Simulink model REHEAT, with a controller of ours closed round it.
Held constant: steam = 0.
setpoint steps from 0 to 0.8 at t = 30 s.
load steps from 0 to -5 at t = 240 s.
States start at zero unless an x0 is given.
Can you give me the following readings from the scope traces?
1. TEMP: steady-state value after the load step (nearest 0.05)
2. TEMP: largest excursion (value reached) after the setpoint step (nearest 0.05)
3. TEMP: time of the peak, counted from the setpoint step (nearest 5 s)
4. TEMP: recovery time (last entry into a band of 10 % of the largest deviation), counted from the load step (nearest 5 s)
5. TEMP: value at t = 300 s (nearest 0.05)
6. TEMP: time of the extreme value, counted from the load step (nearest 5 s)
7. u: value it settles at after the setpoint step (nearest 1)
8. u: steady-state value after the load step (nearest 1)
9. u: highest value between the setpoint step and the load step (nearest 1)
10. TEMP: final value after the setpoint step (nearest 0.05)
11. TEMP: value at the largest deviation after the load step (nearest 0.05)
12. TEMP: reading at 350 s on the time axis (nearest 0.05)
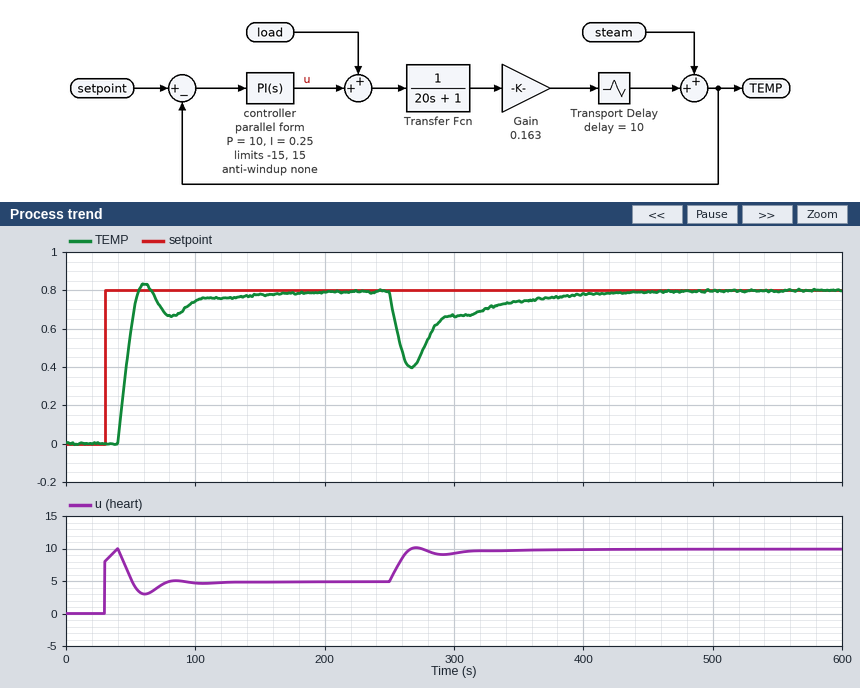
0.80
0.85
30 s
130 s
0.65
25 s
5
10
10
0.80
0.40
0.75
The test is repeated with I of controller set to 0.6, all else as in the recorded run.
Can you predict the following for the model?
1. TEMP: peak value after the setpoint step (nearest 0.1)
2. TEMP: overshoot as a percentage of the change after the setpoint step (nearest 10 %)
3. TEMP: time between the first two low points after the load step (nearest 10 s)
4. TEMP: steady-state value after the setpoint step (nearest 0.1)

1.1
40 %
60 s
0.8
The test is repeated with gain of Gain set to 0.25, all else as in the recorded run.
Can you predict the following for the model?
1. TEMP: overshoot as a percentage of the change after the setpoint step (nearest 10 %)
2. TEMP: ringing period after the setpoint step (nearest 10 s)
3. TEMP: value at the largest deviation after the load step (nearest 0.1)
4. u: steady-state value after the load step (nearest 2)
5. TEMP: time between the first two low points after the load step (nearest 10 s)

40 %
40 s
0.2
8
40 s
